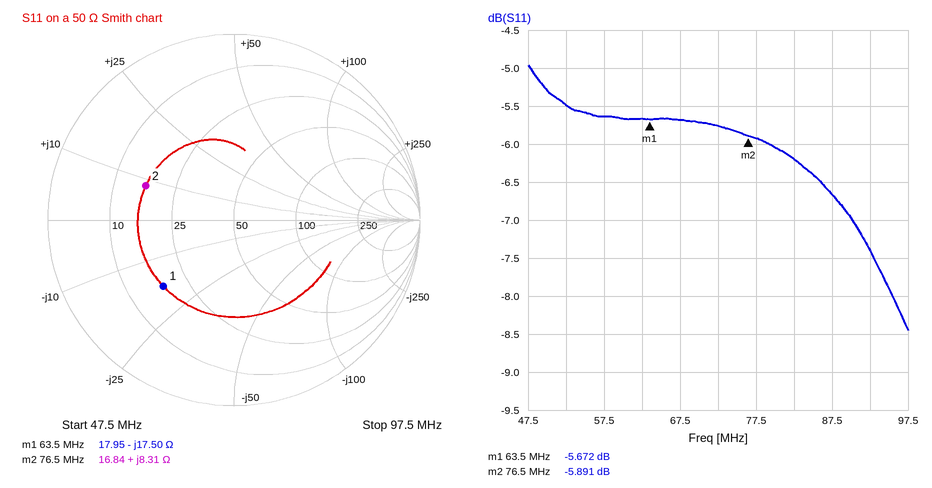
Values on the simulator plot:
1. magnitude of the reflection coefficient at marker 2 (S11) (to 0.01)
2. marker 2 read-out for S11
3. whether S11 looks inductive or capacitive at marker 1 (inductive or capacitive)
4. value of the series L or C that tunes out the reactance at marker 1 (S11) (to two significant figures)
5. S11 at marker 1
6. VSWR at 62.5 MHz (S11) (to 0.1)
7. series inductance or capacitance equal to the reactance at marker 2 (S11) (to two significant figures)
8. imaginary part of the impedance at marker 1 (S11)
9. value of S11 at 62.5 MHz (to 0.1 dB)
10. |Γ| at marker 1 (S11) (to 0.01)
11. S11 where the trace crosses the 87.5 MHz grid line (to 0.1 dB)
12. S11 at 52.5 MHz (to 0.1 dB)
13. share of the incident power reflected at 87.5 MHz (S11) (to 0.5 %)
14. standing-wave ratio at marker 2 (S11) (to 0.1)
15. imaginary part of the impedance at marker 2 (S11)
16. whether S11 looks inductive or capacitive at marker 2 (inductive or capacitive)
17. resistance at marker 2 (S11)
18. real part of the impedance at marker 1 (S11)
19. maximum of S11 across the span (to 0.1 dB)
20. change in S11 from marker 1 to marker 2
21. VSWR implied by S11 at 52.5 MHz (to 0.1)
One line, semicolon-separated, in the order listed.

0.51; -5.891 dB; capacitive; 44 nH; -5.672 dB; 3.2; 17 nH; -17.50 Ω; -5.7 dB; 0.52; -6.7 dB; -5.5 dB; 21.5 %; 3.1; +8.31 Ω; inductive; 16.84 Ω; 17.95 Ω; -5.0 dB; -0.219 dB; 3.3
